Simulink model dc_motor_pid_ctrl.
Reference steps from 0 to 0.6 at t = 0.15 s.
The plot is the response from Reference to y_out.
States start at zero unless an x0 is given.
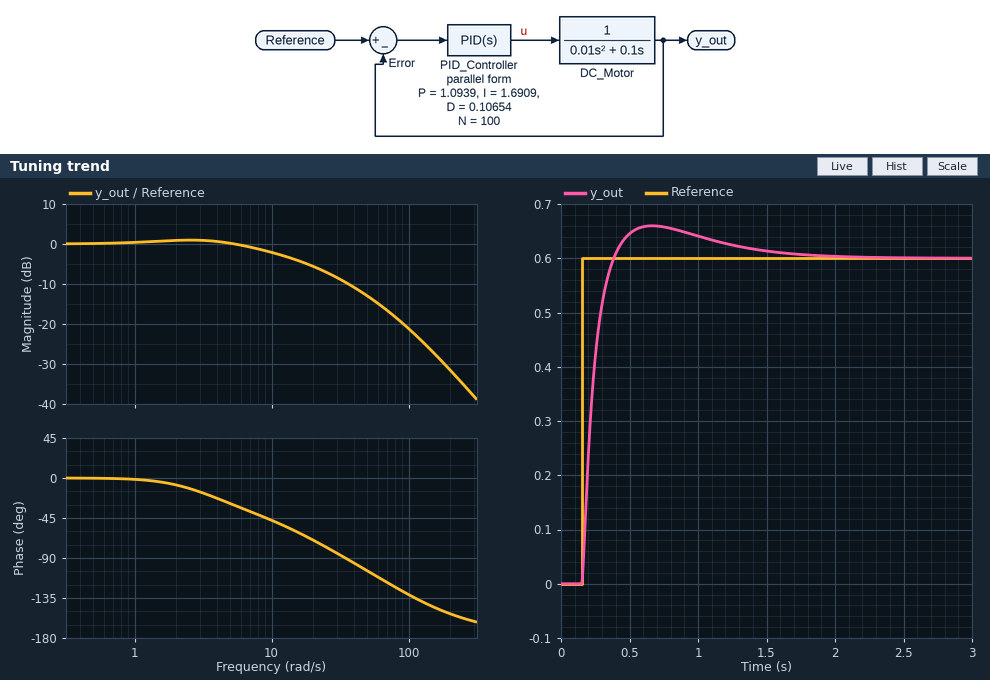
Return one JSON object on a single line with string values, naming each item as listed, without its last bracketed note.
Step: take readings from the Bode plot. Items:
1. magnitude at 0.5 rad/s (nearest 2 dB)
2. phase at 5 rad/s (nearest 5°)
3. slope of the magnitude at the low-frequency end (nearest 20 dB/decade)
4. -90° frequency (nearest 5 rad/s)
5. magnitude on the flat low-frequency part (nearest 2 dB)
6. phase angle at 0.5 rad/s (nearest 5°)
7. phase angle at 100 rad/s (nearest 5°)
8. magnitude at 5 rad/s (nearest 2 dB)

{"magnitude at 0.5 rad/s": "0 dB", "phase at 5 rad/s": "-30°", "slope of the magnitude at the low-frequency end": "0 dB/decade", "-90° frequency": "35 rad/s", "magnitude on the flat low-frequency part": "0 dB", "phase angle at 0.5 rad/s": "0°", "phase angle at 100 rad/s": "-130°", "magnitude at 5 rad/s": "0 dB"}
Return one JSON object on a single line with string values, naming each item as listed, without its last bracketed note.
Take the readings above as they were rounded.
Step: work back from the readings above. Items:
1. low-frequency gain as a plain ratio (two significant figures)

{"low-frequency gain as a plain ratio": "1.0"}
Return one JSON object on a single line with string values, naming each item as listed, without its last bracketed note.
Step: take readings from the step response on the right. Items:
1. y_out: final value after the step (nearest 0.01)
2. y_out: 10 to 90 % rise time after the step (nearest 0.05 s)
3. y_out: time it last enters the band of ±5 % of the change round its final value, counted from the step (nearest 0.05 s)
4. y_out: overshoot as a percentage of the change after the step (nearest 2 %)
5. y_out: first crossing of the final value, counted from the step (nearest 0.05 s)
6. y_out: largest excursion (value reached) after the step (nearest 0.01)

{"y_out: final value after the step": "0.60", "y_out: 10 to 90 % rise time after the step": "0.15 s", "y_out: time it last enters the band of ±5 % of the change round its final value, counted from the step": "1.00 s", "y_out: overshoot as a percentage of the change after the step": "10 %", "y_out: first crossing of the final value, counted from the step": "0.25 s", "y_out: largest excursion (value reached) after the step": "0.66"}
